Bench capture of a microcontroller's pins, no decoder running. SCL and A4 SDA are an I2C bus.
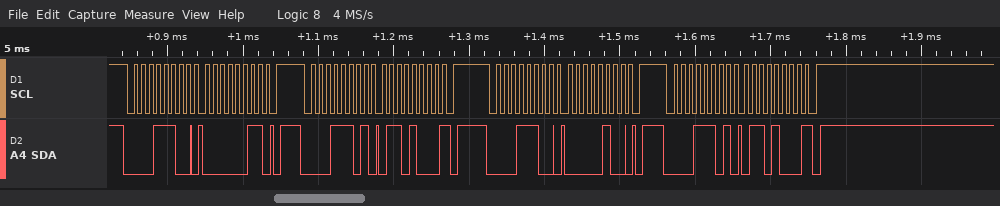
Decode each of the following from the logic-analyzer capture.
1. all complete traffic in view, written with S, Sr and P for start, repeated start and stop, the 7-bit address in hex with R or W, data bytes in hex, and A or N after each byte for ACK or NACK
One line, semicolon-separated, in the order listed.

S 0EW A 03 A P S 0ER A 68 N P S 0EW A 04 A P S 0ER A 68 N P
